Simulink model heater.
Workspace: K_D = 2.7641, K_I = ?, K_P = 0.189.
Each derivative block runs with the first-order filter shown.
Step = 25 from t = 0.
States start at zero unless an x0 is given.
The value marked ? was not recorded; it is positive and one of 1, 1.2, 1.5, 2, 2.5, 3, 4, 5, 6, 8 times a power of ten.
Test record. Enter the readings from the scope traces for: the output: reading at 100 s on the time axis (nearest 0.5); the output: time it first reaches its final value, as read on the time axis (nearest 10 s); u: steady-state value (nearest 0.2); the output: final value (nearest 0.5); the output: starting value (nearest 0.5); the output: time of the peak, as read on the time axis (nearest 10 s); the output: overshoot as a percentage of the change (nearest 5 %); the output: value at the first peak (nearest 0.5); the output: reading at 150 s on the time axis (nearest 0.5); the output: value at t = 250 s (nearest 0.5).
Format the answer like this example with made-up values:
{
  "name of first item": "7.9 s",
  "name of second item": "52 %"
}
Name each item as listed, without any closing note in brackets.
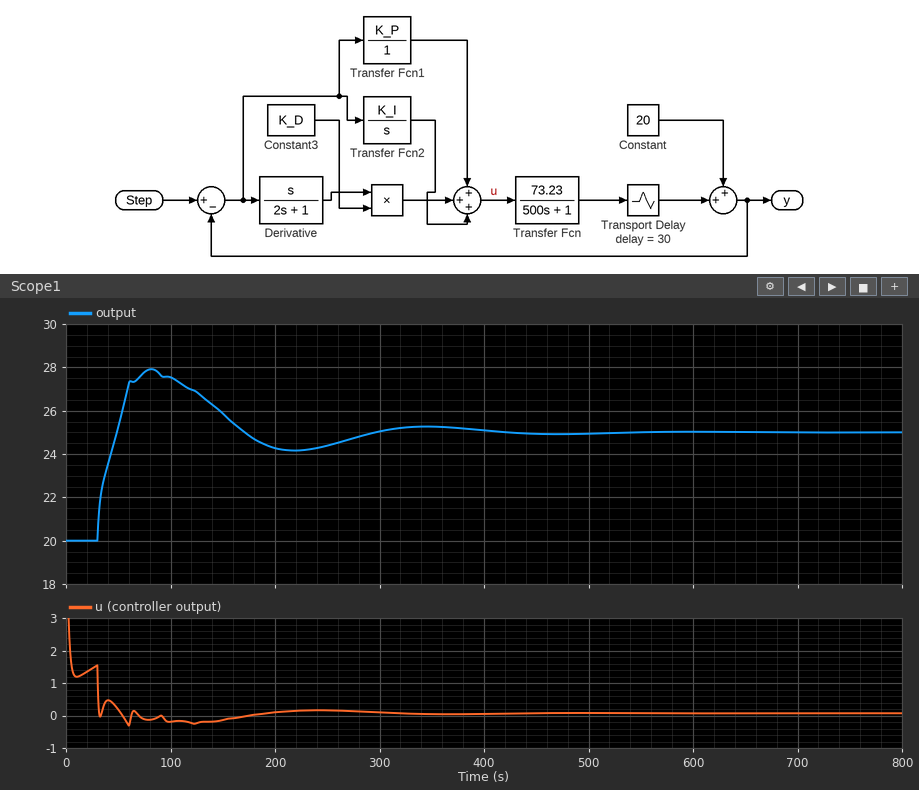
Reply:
{
  "the output: reading at 100 s on the time axis": "27.5",
  "the output: time it first reaches its final value, as read on the time axis": "50 s",
  "u: steady-state value": "0.0",
  "the output: final value": "25.0",
  "the output: starting value": "20.0",
  "the output: time of the peak, as read on the time axis": "80 s",
  "the output: overshoot as a percentage of the change": "60 %",
  "the output: value at the first peak": "28.0",
  "the output: reading at 150 s on the time axis": "26.0",
  "the output: value at t = 250 s": "24.5"
}
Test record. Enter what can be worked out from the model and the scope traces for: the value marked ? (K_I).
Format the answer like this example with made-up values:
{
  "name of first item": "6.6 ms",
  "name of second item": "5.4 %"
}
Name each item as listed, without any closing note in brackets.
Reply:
{
  "the value marked ?": "0.004"
}
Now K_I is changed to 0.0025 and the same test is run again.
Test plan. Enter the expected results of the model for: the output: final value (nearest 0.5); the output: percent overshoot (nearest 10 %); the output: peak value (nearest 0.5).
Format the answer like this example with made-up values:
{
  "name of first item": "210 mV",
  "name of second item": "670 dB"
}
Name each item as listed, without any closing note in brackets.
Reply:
{
  "the output: final value": "25.0",
  "the output: percent overshoot": "40 %",
  "the output: peak value": "27.0"
}
